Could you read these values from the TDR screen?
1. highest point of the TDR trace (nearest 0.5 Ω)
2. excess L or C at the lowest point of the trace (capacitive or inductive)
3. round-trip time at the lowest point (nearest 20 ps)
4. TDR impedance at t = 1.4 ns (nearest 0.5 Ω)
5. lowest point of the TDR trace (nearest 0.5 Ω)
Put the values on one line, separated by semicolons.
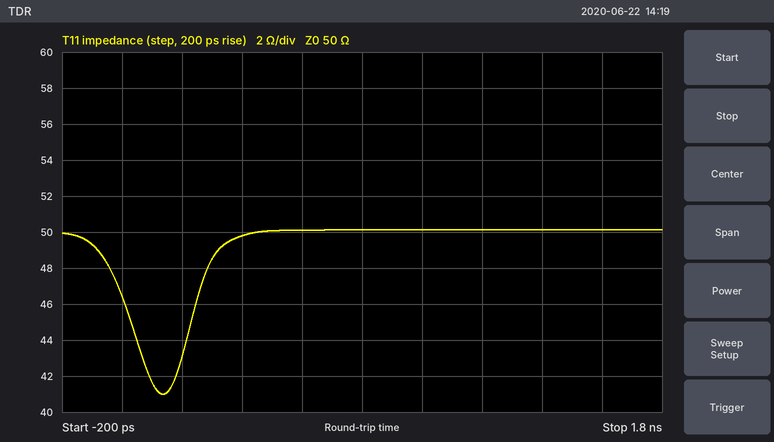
50.0 Ω; capacitive; 140 ps; 50.0 Ω; 41.0 Ω
